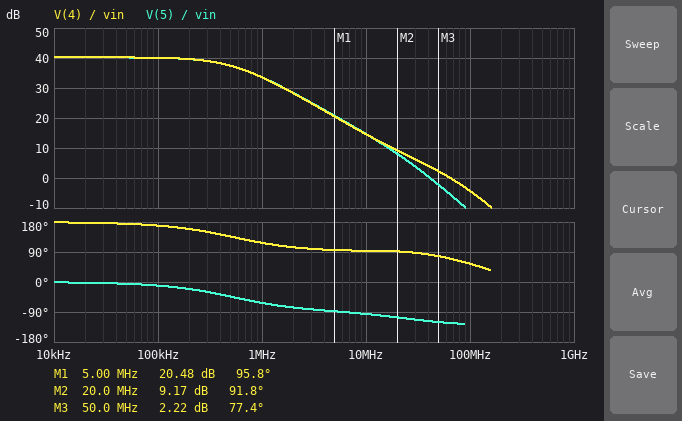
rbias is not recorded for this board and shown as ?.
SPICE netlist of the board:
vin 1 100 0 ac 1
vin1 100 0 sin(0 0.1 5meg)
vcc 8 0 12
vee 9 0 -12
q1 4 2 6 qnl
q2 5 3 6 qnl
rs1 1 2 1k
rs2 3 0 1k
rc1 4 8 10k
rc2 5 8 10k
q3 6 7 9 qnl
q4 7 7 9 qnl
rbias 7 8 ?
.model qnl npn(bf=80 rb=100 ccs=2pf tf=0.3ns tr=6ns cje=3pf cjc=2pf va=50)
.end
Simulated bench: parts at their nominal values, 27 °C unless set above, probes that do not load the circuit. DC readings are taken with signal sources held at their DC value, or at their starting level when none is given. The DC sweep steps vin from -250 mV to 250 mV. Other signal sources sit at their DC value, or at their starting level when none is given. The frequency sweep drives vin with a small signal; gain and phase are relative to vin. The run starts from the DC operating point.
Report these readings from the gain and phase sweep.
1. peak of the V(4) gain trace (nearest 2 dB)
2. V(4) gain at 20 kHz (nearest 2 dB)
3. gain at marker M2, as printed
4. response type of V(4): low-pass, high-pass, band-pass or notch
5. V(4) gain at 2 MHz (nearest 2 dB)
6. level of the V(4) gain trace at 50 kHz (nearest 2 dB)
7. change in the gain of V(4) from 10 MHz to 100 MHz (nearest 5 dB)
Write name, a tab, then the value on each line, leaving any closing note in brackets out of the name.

peak of the V(4) gain trace	40 dB
V(4) gain at 20 kHz	40 dB
gain at marker M2, as printed	9.17 dB
response type of V(4): low-pass, high-pass, band-pass or notch	low-pass
V(4) gain at 2 MHz	28 dB
level of the V(4) gain trace at 50 kHz	40 dB
change in the gain of V(4) from 10 MHz to 100 MHz	-20 dB
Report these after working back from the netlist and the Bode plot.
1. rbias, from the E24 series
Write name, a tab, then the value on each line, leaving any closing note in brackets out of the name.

rbias, from the E24 series	15 kΩ
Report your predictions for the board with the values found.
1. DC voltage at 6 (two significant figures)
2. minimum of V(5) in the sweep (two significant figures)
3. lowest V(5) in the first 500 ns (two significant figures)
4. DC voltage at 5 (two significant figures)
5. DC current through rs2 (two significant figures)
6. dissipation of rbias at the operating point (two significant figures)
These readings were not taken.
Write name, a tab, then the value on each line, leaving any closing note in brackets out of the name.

DC voltage at 6	-780 mV
minimum of V(5) in the sweep	-940 mV
lowest V(5) in the first 500 ns	2.2 V
DC voltage at 5	3.0 V
DC current through rs2	11 µA
dissipation of rbias at the operating point	36 mW
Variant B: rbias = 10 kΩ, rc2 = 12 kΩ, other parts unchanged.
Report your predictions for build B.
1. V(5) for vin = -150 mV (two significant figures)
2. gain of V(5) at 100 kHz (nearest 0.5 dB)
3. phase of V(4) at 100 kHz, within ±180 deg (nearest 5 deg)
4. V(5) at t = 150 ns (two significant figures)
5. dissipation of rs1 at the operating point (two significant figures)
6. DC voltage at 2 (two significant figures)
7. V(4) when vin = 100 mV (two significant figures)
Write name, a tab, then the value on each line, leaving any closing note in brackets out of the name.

V(5) for vin = -150 mV	-1.0 V
gain of V(5) at 100 kHz	-6.0 dB
phase of V(4) at 100 kHz, within ±180 deg	0 deg
V(5) at t = 150 ns	-970 mV
dissipation of rs1 at the operating point	31 µW
DC voltage at 2	-180 mV
V(4) when vin = 100 mV	-880 mV
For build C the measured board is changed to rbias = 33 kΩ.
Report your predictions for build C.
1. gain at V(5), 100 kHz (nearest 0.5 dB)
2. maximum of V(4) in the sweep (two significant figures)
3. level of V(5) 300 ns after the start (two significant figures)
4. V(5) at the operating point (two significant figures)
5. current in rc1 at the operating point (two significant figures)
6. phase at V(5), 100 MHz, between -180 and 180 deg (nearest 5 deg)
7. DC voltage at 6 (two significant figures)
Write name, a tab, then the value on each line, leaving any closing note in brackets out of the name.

gain at V(5), 100 kHz	36.0 dB
maximum of V(4) in the sweep	12 V
level of V(5) 300 ns after the start	9.3 V
V(5) at the operating point	7.9 V
current in rc1 at the operating point	410 µA
phase at V(5), 100 MHz, between -180 and 180 deg	-150 deg
DC voltage at 6	-750 mV
